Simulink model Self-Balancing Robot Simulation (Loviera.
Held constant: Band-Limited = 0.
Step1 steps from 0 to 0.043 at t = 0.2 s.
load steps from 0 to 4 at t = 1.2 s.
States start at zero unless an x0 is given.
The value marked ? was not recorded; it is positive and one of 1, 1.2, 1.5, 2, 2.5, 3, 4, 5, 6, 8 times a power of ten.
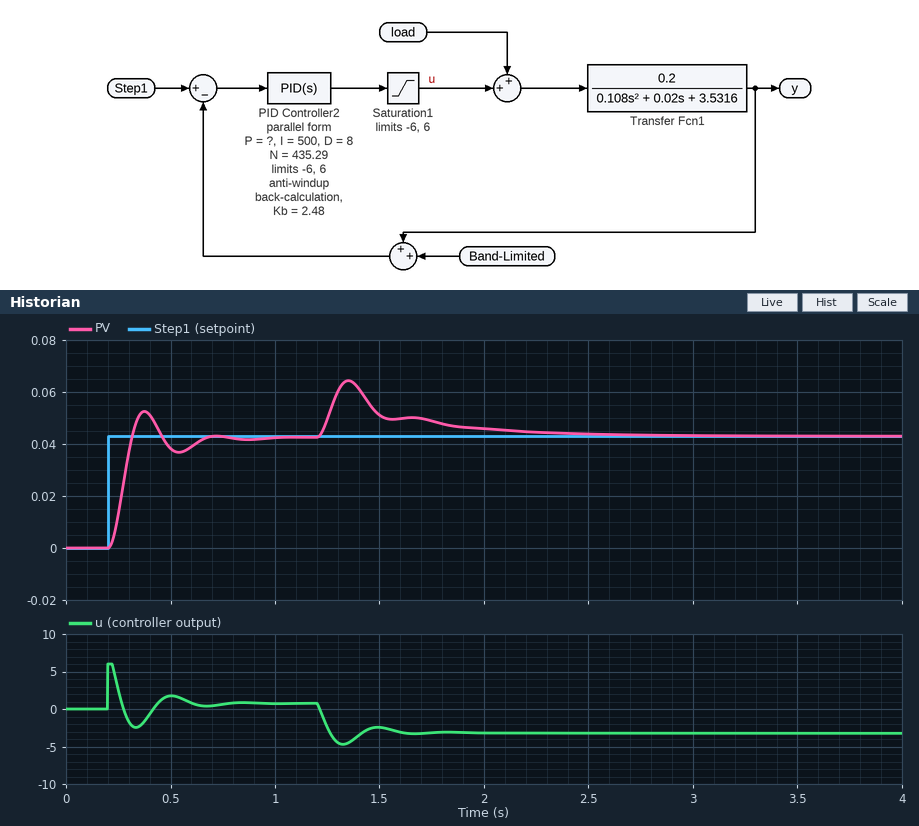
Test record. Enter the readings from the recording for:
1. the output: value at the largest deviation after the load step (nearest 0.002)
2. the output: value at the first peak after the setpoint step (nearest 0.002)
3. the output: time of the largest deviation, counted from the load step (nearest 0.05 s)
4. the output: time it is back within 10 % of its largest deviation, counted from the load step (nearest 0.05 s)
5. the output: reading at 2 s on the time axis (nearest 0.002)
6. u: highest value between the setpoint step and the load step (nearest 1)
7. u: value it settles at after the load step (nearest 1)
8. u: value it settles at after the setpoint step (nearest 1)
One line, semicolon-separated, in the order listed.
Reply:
0.064; 0.052; 0.15 s; 0.90 s; 0.046; 6; -3; 1
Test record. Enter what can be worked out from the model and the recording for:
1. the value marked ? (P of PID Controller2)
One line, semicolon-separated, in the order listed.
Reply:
200
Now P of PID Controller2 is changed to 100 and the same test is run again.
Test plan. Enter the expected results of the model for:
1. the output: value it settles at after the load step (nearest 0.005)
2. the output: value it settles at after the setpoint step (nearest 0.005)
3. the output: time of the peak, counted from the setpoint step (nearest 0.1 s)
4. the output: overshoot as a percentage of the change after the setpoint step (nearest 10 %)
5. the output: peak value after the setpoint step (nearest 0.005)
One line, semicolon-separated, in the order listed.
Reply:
0.045; 0.045; 0.3 s; 20 %; 0.050
